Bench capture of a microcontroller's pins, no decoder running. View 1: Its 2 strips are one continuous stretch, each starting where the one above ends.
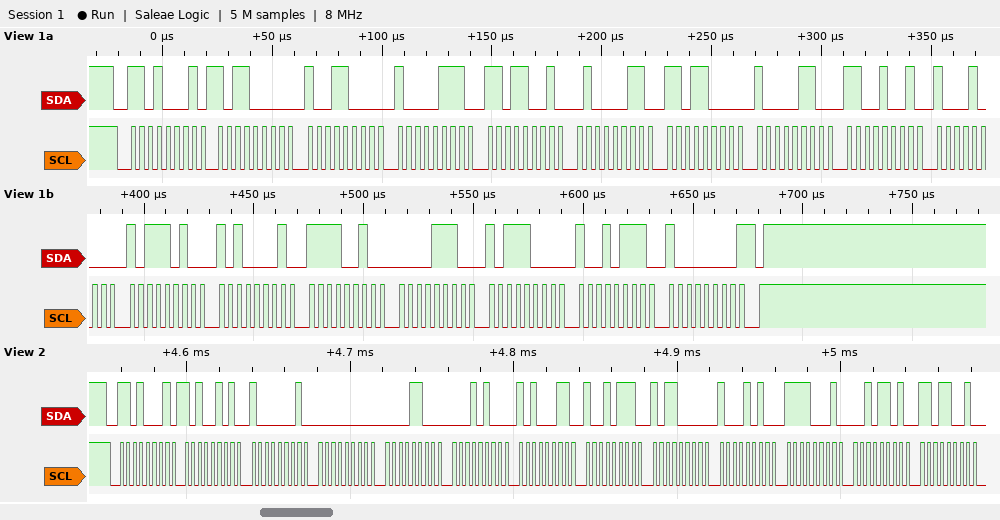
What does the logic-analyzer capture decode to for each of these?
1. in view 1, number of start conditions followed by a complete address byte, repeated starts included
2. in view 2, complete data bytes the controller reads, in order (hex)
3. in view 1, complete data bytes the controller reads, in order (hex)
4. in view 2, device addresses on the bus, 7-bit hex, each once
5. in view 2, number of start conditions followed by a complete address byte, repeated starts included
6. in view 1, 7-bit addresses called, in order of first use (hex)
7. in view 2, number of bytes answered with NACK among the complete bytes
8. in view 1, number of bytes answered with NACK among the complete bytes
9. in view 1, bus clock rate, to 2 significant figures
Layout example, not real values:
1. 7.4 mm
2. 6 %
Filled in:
1. 1
2. A5 81 00 0C 14 A3 97 B0 8A F1 2D D9
3. B0 98 87 D9 43 D8 86 C9 88 BA A1 F2 0E B8 97 80
4. 0x68
5. 1
6. 0x68
7. 0
8. 1
9. 250 kHz
